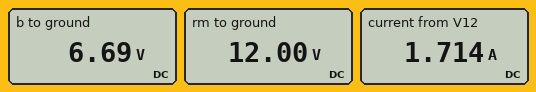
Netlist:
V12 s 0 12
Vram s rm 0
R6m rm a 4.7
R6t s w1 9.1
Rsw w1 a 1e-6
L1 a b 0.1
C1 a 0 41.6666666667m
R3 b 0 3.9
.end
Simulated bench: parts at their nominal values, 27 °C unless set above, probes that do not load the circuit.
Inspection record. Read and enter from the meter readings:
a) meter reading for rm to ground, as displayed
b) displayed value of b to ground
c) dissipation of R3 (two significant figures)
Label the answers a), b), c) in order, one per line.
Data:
a) 12.00 V
b) 6.69 V
c) 11 W
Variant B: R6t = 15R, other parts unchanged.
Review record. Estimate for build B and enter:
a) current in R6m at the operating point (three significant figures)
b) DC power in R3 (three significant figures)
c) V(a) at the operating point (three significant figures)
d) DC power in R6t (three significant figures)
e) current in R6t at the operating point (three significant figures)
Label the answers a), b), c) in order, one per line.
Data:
a) 1.22 A
b) 10.0 W
c) 6.26 V
d) 2.20 W
e) 383 mA
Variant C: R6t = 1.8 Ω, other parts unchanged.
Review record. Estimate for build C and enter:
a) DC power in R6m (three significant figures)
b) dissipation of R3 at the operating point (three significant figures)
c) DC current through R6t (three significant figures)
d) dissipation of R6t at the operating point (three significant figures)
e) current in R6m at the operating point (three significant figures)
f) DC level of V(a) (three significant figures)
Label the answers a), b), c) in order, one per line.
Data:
a) 1.92 W
b) 20.8 W
c) 1.67 A
d) 5.01 W
e) 639 mA
f) 9.00 V
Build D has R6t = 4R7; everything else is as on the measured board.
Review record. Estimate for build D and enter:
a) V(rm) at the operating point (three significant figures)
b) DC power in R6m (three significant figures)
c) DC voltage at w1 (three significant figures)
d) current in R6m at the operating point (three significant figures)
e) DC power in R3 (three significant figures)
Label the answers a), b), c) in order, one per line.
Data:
a) 12.0 V
b) 4.33 W
c) 7.49 V
d) 960 mA
e) 14.4 W
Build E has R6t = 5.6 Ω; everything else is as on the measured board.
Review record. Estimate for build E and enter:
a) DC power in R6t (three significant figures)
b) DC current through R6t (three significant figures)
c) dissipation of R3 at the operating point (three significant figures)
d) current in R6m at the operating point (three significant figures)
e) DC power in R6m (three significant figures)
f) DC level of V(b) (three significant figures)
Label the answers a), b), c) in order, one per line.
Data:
a) 4.03 W
b) 848 mA
c) 13.5 W
d) 1.01 A
e) 4.80 W
f) 7.25 V
